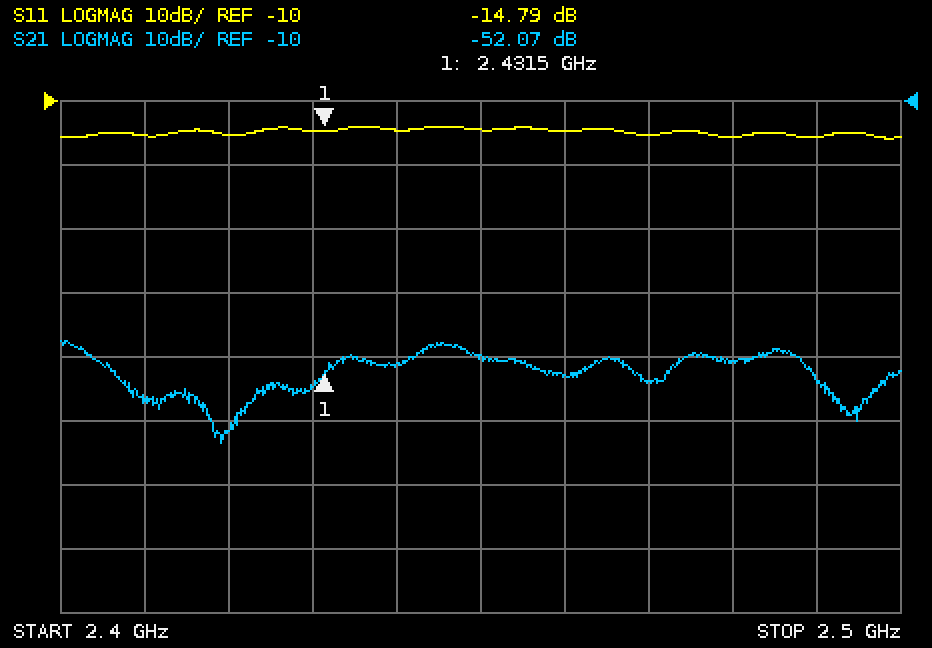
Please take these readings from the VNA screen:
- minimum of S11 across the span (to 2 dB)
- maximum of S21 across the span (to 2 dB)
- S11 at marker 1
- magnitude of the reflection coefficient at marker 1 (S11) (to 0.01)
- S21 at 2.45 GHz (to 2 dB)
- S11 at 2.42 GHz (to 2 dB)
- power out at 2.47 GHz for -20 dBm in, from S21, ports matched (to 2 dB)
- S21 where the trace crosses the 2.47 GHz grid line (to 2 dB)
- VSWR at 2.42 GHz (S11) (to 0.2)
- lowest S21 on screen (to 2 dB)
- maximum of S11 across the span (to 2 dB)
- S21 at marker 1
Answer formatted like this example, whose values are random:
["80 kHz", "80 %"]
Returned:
["-16 dB", "-48 dB", "-14.79 dB", "0.18", "-50 dB", "-16 dB", "-74 dBm", "-54 dB", "1.4", "-64 dB", "-14 dB", "-52.07 dB"]
